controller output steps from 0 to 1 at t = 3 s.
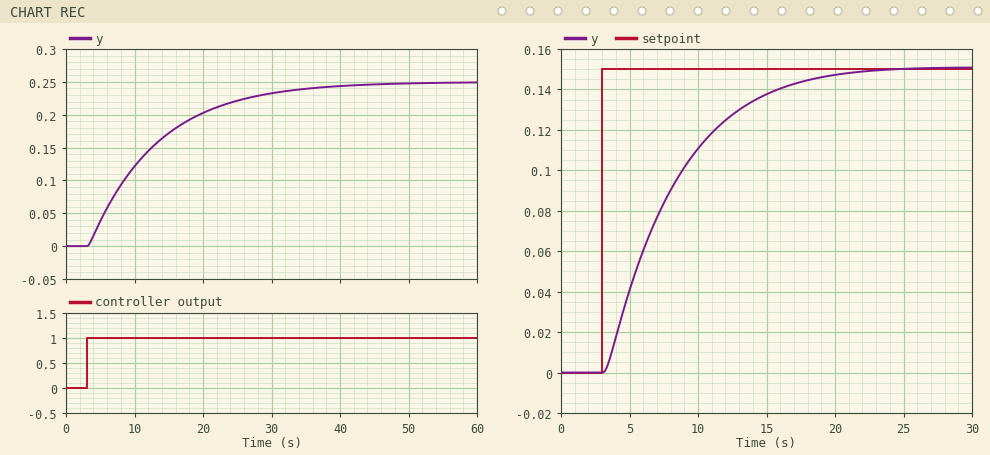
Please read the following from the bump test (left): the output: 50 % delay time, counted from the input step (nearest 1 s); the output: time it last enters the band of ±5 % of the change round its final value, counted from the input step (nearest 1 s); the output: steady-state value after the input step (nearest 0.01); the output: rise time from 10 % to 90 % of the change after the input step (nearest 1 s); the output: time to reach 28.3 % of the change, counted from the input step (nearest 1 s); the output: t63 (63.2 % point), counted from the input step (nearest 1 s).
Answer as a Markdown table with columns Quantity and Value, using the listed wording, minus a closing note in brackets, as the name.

| Quantity | Value |
|---|---|
| the output: 50 % delay time, counted from the input step | 7 s |
| the output: time it last enters the band of ±5 % of the change round its final value, counted from the input step | 30 s |
| the output: steady-state value after the input step | 0.25 |
| the output: rise time from 10 % to 90 % of the change after the input step | 22 s |
| the output: time to reach 28.3 % of the change, counted from the input step | 4 s |
| the output: t63 (63.2 % point), counted from the input step | 10 s |
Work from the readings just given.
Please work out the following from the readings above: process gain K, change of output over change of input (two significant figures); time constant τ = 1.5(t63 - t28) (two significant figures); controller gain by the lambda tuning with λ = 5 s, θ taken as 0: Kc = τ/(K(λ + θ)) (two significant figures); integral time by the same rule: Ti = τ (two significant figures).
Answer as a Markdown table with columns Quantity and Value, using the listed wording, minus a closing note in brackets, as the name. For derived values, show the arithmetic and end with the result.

| Quantity | Value |
|---|---|
| process gain K, change of output over change of input | (0.25 - 0) / 1 = 0.25 |
| time constant τ = 1.5(t63 - t28) | 1.5 × (10 - 4) = 9.0 s |
| controller gain by the lambda tuning with λ = 5 s, θ taken as 0: Kc = τ/(K(λ + θ)) | 9 / (0.25 × (5 + 0)) = 7.2 |
| integral time by the same rule: Ti = τ | 9.0 s |
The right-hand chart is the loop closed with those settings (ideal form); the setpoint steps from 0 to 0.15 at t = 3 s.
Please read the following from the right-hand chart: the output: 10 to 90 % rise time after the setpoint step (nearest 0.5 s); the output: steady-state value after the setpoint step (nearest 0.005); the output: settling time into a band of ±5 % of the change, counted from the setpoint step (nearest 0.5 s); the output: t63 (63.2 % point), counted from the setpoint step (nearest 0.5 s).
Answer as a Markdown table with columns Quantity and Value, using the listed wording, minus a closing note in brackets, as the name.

| Quantity | Value |
|---|---|
| the output: 10 to 90 % rise time after the setpoint step | 10.5 s |
| the output: steady-state value after the setpoint step | 0.150 |
| the output: settling time into a band of ±5 % of the change, counted from the setpoint step | 14.0 s |
| the output: t63 (63.2 % point), counted from the setpoint step | 5.5 s |
